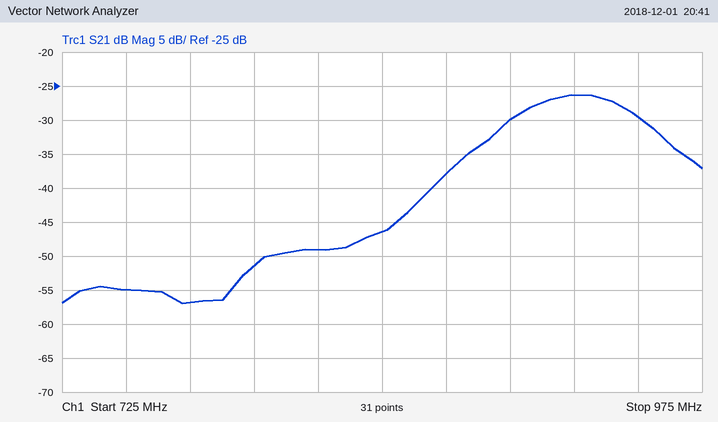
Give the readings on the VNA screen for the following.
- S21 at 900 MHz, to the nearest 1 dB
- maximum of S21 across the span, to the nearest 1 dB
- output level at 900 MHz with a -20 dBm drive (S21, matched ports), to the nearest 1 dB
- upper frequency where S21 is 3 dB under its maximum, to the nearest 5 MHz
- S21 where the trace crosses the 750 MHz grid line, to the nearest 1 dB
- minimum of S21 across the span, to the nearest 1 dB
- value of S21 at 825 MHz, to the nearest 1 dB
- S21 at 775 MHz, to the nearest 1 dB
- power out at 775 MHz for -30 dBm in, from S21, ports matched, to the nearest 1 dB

-30 dB
-26 dB
-50 dBm
950 MHz
-55 dB
-57 dB
-49 dB
-57 dB
-87 dBm
